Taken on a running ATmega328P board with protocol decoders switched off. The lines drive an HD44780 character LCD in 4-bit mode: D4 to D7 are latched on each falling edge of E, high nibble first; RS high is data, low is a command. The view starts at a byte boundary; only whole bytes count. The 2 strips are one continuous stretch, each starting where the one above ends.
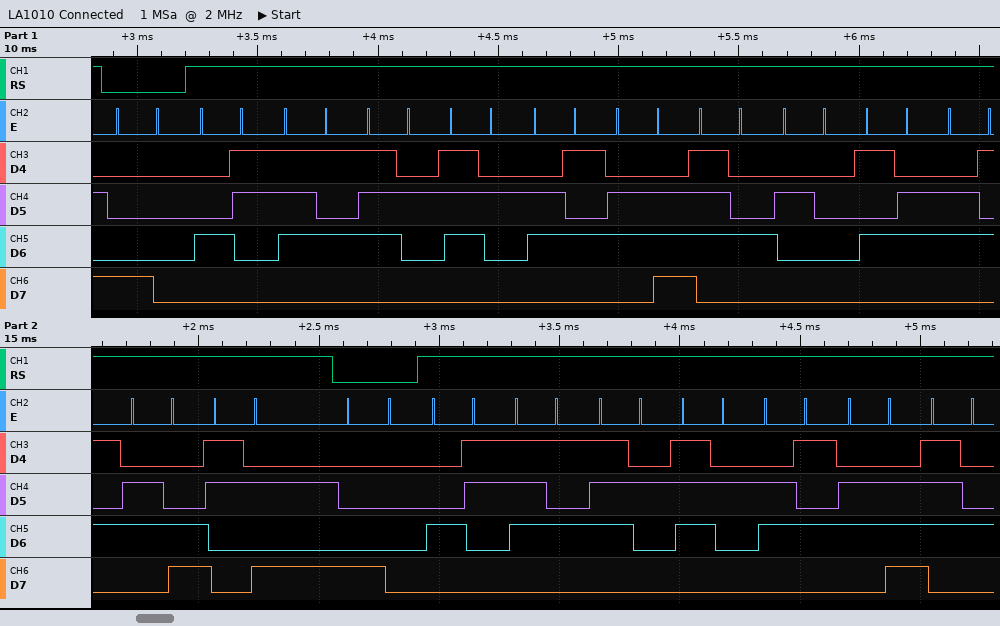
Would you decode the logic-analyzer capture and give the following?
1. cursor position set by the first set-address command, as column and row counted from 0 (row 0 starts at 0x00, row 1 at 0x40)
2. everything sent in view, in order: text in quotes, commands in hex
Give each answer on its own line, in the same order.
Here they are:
column 0, row 0
0x80 "Current Vel:" 0x80 "Current"
